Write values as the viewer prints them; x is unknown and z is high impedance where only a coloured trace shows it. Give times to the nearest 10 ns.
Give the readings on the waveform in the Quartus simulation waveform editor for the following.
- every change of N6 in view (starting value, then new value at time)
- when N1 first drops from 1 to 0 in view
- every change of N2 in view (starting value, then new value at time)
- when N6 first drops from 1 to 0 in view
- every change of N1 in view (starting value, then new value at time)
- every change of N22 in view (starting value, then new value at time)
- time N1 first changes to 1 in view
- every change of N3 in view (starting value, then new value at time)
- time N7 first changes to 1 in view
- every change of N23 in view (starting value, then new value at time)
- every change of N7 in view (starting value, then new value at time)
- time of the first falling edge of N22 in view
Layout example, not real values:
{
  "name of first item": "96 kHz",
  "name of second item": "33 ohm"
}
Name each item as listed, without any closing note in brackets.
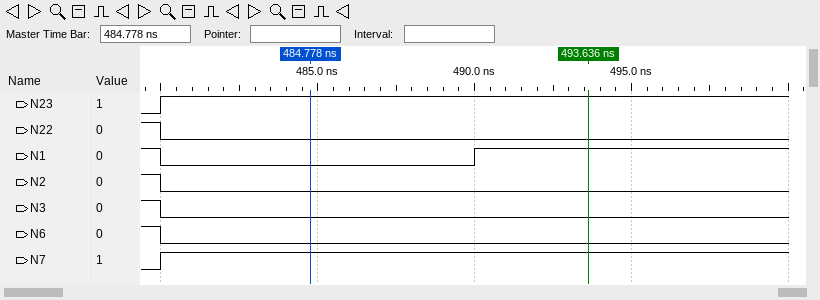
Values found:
{
  "every change of N6 in view": "1, 0 at 480 ns",
  "when N1 first drops from 1 to 0 in view": "480 ns",
  "every change of N2 in view": "1, 0 at 480 ns",
  "when N6 first drops from 1 to 0 in view": "480 ns",
  "every change of N1 in view": "1, 0 at 480 ns, 1 at 490 ns",
  "every change of N22 in view": "1, 0 at 480 ns",
  "time N1 first changes to 1 in view": "490 ns",
  "every change of N3 in view": "1, 0 at 480 ns",
  "time N7 first changes to 1 in view": "480 ns",
  "every change of N23 in view": "0, 1 at 480 ns",
  "every change of N7 in view": "0, 1 at 480 ns",
  "time of the first falling edge of N22 in view": "480 ns"
}
